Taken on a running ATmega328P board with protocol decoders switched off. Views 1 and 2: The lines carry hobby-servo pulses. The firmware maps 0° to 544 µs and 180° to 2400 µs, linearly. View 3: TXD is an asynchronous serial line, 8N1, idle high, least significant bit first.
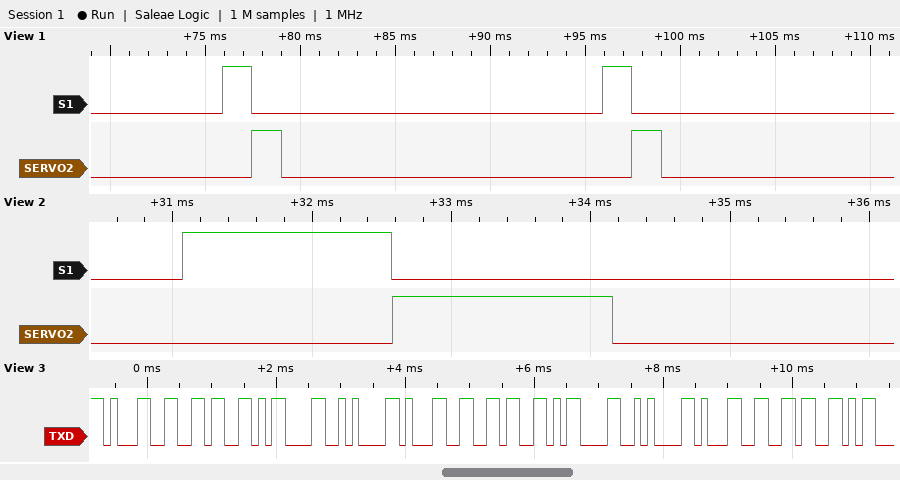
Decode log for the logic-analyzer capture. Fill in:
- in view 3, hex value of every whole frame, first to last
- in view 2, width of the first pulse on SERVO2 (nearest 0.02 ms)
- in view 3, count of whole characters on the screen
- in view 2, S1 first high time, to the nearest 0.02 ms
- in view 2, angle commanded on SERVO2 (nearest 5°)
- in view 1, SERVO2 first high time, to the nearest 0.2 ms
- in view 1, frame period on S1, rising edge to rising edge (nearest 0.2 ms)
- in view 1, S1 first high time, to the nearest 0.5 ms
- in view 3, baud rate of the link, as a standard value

0x31 0x36 0x0D 0x0A 0x31 0x36 0x0D 0x0A 0x31 0x36
1.58 ms
10
1.50 ms
100°
1.6 ms
20.0 ms
1.5 ms
9600 baud
